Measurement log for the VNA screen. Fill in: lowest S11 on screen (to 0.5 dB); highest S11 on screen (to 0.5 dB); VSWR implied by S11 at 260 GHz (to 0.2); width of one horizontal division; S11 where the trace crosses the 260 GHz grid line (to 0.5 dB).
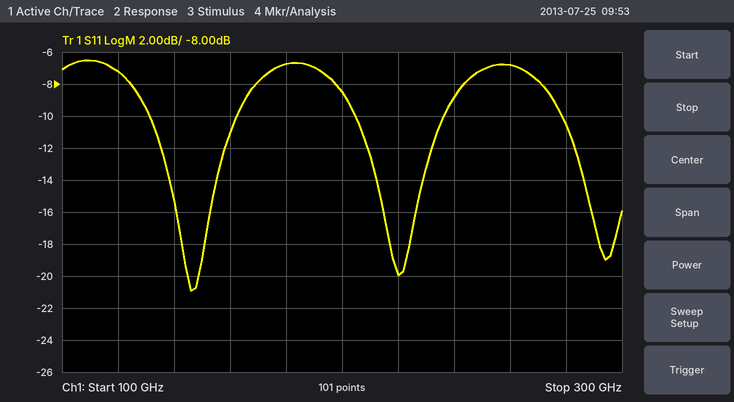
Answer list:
-21.0 dB
-6.5 dB
2.6
20 GHz
-7.0 dB
